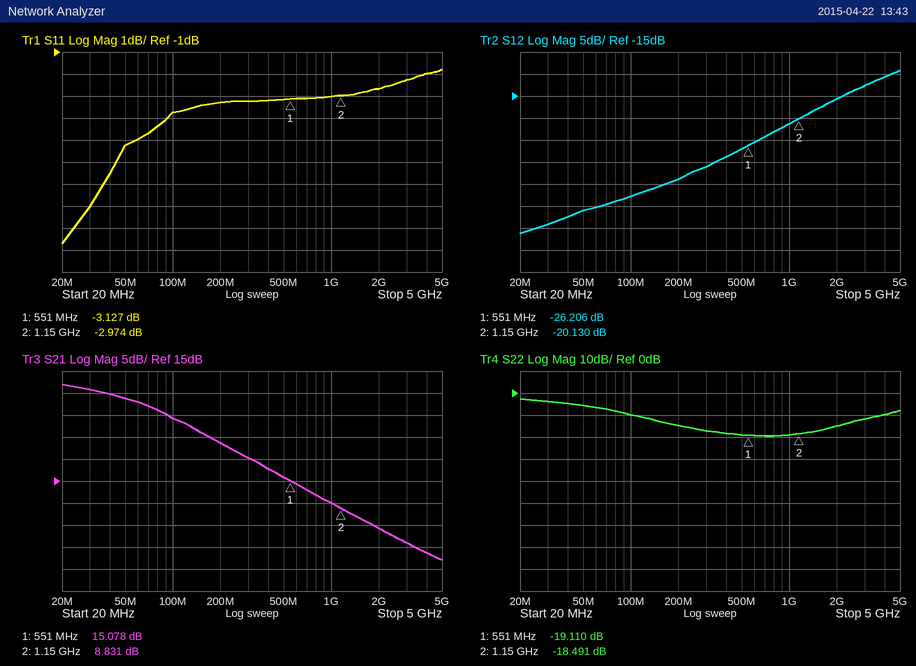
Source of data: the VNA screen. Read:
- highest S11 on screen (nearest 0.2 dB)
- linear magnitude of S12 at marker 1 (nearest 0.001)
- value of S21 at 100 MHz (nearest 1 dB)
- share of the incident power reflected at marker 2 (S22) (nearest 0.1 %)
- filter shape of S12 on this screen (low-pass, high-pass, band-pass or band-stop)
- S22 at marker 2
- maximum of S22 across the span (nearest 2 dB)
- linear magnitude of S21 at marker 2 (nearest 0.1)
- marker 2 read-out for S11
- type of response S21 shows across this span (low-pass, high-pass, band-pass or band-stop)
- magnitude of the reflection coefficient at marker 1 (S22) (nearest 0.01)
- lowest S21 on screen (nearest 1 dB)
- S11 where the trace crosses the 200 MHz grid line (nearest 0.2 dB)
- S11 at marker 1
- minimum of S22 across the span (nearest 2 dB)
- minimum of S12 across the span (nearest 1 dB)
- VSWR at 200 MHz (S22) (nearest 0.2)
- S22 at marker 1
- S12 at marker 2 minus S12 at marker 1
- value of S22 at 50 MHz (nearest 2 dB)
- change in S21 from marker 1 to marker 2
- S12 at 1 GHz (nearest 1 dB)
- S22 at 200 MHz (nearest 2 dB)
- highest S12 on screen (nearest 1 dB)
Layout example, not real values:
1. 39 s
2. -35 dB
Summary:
1. -1.8 dB
2. 0.049
3. 29 dB
4. 1.4 %
5. high-pass
6. -18.491 dB
7. -2 dB
8. 2.8
9. -2.974 dB
10. low-pass
11. 0.11
12. -3 dB
13. -3.2 dB
14. -3.127 dB
15. -20 dB
16. -46 dB
17. 1.4
18. -19.110 dB
19. 6.076 dB
20. -6 dB
21. -6.247 dB
22. -21 dB
23. -14 dB
24. -9 dB
